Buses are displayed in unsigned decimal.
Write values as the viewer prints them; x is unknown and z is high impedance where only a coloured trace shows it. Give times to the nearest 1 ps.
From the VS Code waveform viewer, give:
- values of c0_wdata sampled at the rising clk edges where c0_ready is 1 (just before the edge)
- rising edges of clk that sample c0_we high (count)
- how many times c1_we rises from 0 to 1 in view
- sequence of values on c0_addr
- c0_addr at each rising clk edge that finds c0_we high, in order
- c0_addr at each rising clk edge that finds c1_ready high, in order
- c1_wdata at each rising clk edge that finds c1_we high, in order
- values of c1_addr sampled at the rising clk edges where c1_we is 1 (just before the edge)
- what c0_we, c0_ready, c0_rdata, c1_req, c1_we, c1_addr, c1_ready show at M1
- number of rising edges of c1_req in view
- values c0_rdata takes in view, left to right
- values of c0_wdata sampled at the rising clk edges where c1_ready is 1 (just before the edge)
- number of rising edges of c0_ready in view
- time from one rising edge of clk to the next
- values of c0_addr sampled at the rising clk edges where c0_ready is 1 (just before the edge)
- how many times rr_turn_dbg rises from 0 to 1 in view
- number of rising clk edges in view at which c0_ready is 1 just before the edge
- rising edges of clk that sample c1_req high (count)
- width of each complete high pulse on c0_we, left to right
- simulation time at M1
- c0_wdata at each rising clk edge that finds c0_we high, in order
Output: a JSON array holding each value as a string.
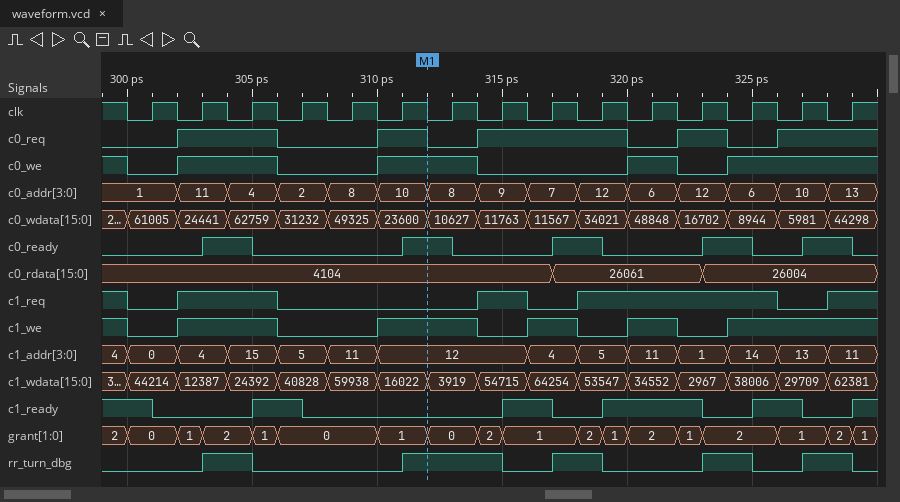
["62759, 10627, 34021, 8944, 44298", "8", "5", "1, 11, 4, 2, 8, 10, 8, 9, 7, 12, 6, 12, 6, 10, 13", "11, 4, 10, 8, 6, 6, 10, 13", "1, 2, 7, 6, 12, 10", "12387, 24392, 16022, 3919, 64254, 34552, 38006, 29709, 62381", "4, 15, 12, 12, 4, 11, 14, 13, 11", "c0_we=1, c0_ready=1, c0_rdata=4104, c1_req=0, c1_we=1, c1_addr=12, c1_ready=0", "4", "4104, 26061, 26004", "61005, 31232, 11567, 48848, 16702, 5981", "5", "2 ps", "4, 8, 12, 6, 13", "5", "5", "8", "4 ps, 4 ps, 2 ps", "312 ps", "24441, 62759, 23600, 10627, 48848, 8944, 5981, 44298"]
